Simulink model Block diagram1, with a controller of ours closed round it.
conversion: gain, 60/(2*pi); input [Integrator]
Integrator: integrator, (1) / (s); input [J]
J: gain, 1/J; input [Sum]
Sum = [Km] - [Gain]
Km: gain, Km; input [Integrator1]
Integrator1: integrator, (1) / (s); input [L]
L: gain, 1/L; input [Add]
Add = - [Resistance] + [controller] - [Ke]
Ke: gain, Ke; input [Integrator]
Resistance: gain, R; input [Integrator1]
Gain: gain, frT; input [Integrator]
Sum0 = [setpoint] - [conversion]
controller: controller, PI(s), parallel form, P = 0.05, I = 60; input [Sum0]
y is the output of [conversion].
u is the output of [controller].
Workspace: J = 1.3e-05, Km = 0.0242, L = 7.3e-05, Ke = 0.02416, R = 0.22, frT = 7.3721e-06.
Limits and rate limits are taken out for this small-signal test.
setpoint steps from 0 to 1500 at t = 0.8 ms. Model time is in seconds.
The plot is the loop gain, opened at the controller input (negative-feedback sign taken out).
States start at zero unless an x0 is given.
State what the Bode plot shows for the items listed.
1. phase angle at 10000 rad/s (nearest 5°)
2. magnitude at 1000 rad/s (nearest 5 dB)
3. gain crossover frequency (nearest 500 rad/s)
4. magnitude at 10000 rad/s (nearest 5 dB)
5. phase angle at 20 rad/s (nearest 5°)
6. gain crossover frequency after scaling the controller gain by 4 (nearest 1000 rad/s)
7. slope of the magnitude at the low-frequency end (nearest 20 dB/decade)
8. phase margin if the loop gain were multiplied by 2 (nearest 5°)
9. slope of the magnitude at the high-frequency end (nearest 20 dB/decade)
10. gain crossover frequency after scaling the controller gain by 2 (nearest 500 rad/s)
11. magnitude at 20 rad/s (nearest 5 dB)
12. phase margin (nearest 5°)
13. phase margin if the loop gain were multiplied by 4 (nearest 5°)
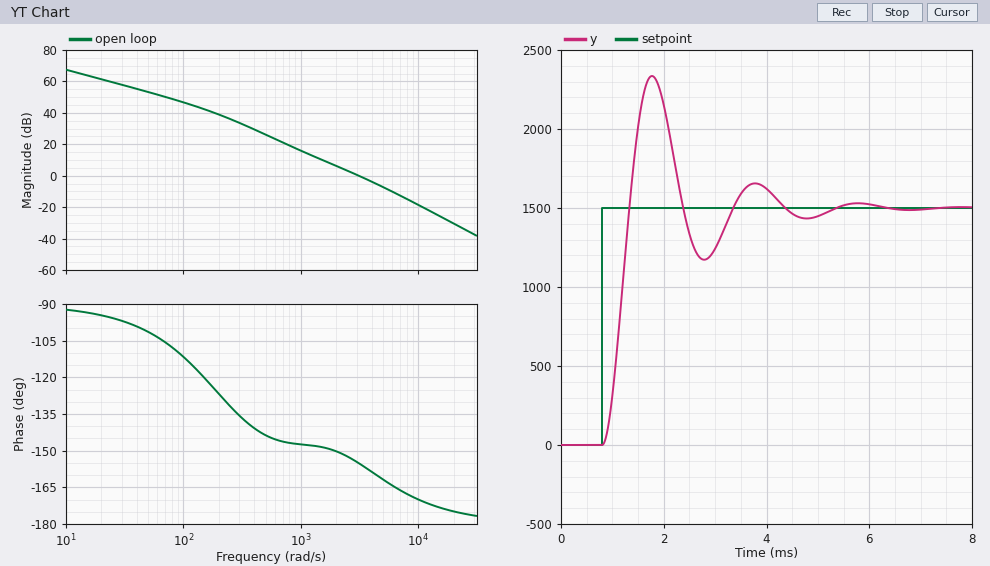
-170°
15 dB
3000 rad/s
-20 dB
-95°
7000 rad/s
-20 dB/decade
20°
-40 dB/decade
4500 rad/s
60 dB
25°
15°
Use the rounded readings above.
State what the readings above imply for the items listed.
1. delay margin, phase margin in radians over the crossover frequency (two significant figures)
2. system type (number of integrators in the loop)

0.00015 s
1
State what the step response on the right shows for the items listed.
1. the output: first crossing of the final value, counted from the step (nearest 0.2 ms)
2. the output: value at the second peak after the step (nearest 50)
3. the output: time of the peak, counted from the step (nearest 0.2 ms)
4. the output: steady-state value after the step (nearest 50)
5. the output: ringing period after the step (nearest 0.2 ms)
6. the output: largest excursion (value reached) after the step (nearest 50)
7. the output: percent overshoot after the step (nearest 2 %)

0.6 ms
1650
1.0 ms
1500
2.0 ms
2350
56 %
